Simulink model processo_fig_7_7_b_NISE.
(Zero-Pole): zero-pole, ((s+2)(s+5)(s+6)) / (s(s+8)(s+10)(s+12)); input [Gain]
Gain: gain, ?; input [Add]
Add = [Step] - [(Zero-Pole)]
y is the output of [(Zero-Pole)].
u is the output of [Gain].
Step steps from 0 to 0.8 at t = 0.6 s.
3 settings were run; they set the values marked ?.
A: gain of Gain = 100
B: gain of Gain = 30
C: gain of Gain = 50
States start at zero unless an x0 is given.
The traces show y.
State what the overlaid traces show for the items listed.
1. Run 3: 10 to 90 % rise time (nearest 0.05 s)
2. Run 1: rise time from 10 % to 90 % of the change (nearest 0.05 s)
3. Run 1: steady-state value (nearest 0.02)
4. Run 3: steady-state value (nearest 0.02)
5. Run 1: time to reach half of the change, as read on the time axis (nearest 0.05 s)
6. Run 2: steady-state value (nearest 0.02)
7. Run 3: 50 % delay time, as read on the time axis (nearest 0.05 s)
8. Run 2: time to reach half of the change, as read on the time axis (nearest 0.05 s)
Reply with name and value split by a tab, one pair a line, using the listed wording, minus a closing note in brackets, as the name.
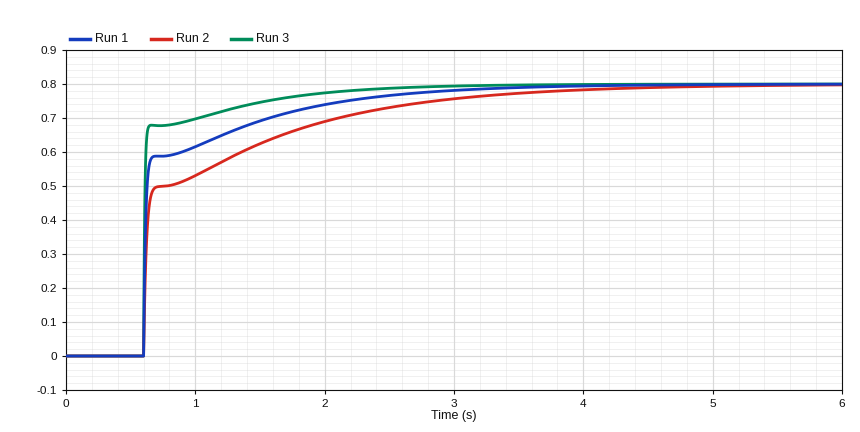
Run 3: 10 to 90 % rise time	0.60 s
Run 1: rise time from 10 % to 90 % of the change	1.15 s
Run 1: steady-state value	0.80
Run 3: steady-state value	0.80
Run 1: time to reach half of the change, as read on the time axis	0.60 s
Run 2: steady-state value	0.80
Run 3: 50 % delay time, as read on the time axis	0.60 s
Run 2: time to reach half of the change, as read on the time axis	0.65 s
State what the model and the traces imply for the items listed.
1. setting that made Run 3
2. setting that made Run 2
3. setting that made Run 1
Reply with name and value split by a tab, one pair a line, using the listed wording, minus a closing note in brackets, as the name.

setting that made Run 3	A
setting that made Run 2	B
setting that made Run 1	C
